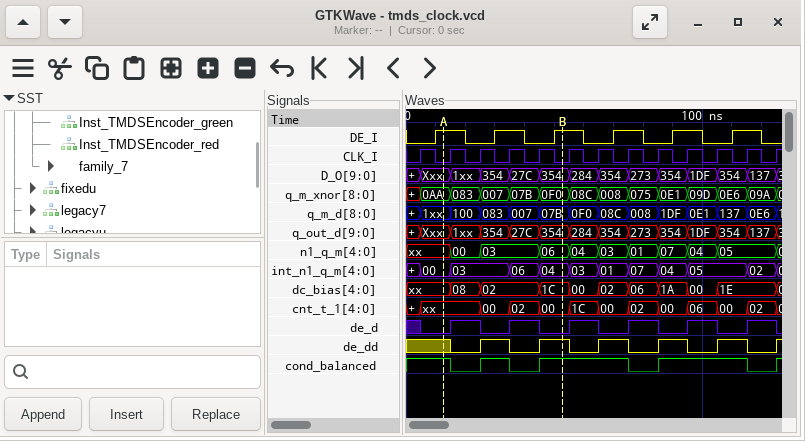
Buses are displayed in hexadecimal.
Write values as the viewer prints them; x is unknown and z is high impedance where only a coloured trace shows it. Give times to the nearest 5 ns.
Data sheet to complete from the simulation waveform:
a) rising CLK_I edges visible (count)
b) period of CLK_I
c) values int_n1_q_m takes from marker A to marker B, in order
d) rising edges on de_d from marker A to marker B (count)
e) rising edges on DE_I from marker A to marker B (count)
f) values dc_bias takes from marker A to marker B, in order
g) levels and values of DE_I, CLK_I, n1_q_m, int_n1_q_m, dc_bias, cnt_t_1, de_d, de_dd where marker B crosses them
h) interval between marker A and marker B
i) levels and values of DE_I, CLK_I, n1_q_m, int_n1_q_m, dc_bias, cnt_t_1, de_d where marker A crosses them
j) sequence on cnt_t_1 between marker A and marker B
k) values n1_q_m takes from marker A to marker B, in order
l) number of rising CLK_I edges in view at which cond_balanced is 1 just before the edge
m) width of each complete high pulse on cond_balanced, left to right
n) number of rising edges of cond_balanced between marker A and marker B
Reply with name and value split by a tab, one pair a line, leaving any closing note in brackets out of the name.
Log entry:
rising CLK_I edges visible	13
period of CLK_I	10 ns
values int_n1_q_m takes from marker A to marker B, in order	00, 03, 06, 04
rising edges on de_d from marker A to marker B	2
rising edges on DE_I from marker A to marker B	2
values dc_bias takes from marker A to marker B, in order	xx, 08, 02, 1C
levels and values of DE_I, CLK_I, n1_q_m, int_n1_q_m, dc_bias, cnt_t_1, de_d, de_dd where marker B crosses them	DE_I=1, CLK_I=0, n1_q_m=06, int_n1_q_m=04, dc_bias=1C, cnt_t_1=00, de_d=0, de_dd=1
interval between marker A and marker B	40 ns
levels and values of DE_I, CLK_I, n1_q_m, int_n1_q_m, dc_bias, cnt_t_1, de_d where marker A crosses them	DE_I=1, CLK_I=0, n1_q_m=xx, int_n1_q_m=00, dc_bias=xx, cnt_t_1=xx, de_d=0
sequence on cnt_t_1 between marker A and marker B	xx, 00, 02, 00
values n1_q_m takes from marker A to marker B, in order	xx, 00, 03, 06
number of rising CLK_I edges in view at which cond_balanced is 1 just before the edge	9
width of each complete high pulse on cond_balanced, left to right	10 ns, 30 ns, 30 ns
number of rising edges of cond_balanced between marker A and marker B	2
